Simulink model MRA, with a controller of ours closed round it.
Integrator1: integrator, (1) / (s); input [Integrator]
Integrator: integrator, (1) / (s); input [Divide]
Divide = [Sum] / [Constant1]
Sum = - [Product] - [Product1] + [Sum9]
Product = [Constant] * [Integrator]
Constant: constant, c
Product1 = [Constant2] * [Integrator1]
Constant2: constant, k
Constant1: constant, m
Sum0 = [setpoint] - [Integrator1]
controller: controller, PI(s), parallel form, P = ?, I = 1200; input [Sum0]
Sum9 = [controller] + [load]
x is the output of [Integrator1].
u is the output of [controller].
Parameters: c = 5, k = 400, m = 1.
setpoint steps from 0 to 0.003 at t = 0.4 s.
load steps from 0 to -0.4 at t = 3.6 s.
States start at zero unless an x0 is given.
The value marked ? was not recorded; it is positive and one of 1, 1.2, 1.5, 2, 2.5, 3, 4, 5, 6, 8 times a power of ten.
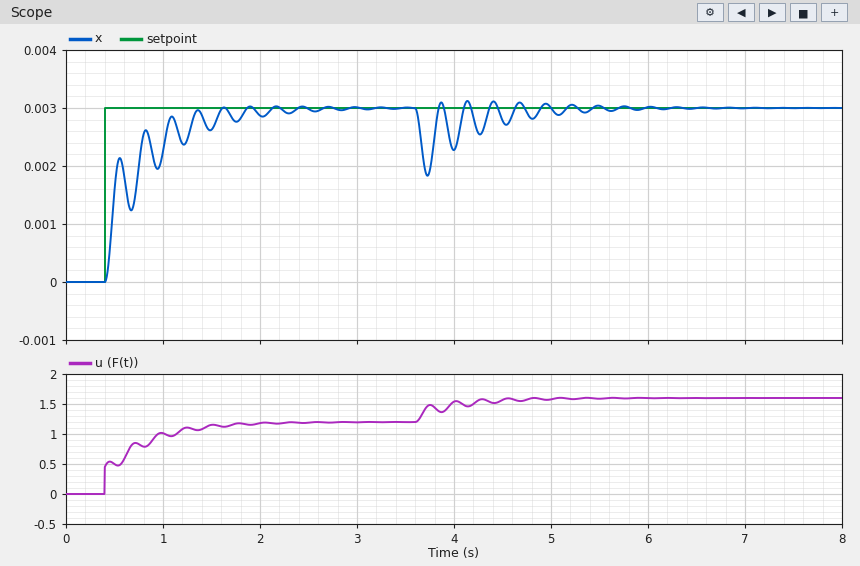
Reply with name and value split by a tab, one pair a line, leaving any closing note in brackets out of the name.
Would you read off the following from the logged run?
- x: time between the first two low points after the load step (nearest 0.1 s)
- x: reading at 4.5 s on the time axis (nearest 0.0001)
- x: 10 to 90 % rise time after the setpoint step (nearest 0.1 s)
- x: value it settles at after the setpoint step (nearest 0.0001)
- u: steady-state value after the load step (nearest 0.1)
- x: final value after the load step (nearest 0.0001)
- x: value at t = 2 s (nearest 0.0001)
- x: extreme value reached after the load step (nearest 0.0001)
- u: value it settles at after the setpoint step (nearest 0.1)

x: time between the first two low points after the load step	0.3 s
x: reading at 4.5 s on the time axis	0.0028
x: 10 to 90 % rise time after the setpoint step	0.6 s
x: value it settles at after the setpoint step	0.0030
u: steady-state value after the load step	1.6
x: final value after the load step	0.0030
x: value at t = 2 s	0.0029
x: extreme value reached after the load step	0.0018
u: value it settles at after the setpoint step	1.2
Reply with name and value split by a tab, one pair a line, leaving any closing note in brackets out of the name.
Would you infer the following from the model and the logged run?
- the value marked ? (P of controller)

the value marked ?	150
